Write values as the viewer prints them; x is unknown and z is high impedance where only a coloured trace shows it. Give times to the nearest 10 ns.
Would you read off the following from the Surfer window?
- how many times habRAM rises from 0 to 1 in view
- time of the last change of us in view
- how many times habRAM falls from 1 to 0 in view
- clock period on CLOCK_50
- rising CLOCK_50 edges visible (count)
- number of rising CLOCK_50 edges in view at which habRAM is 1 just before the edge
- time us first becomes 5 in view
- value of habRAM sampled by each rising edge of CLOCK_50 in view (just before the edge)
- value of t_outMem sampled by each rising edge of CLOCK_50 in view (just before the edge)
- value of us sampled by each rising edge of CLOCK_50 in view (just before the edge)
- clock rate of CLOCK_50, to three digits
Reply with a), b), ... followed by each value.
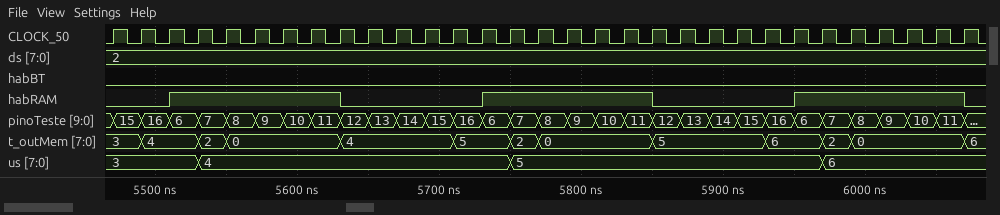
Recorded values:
a) 3
b) 5970 ns
c) 3
d) 20 ns
e) 31
f) 18
g) 5750 ns
h) 0 0 0 1 1 1 1 1 1 0 0 0 0 0 1 1 1 1 1 1 0 0 0 0 0 1 1 1 1 1 1
i) 3, 3, 4, 4, 2, 0, 0, 0, 0, 4, 4, 4, 4, 5, 5, 2, 0, 0, 0, 0, 5, 5, 5, 5, 6, 6, 2, 0, 0, 0, 0
j) 3, 3, 3, 3, 4, 4, 4, 4, 4, 4, 4, 4, 4, 4, 4, 5, 5, 5, 5, 5, 5, 5, 5, 5, 5, 5, 6, 6, 6, 6, 6
k) 50.0 MHz
